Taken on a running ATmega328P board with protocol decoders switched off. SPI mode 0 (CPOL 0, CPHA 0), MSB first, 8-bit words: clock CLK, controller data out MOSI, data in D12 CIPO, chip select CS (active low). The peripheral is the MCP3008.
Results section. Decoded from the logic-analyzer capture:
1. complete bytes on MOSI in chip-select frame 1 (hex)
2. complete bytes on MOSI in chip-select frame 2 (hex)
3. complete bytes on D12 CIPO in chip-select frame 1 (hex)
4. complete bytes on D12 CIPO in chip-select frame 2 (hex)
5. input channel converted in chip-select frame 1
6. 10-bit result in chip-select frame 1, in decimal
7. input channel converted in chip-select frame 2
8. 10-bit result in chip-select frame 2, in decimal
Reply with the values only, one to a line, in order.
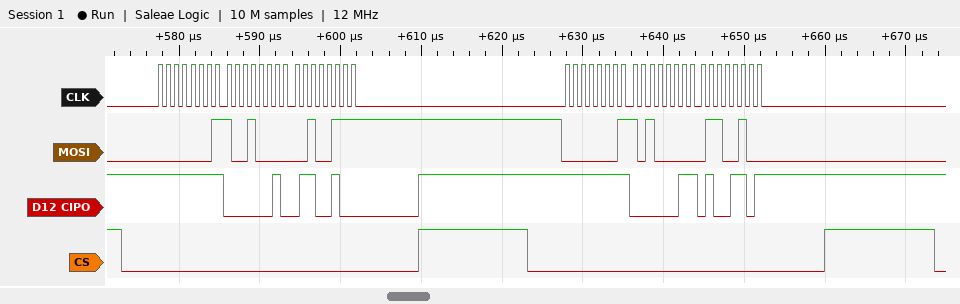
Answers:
01 90 27
01 A0 64
FF 02 64
FF 03 4D
1
612
2
845
